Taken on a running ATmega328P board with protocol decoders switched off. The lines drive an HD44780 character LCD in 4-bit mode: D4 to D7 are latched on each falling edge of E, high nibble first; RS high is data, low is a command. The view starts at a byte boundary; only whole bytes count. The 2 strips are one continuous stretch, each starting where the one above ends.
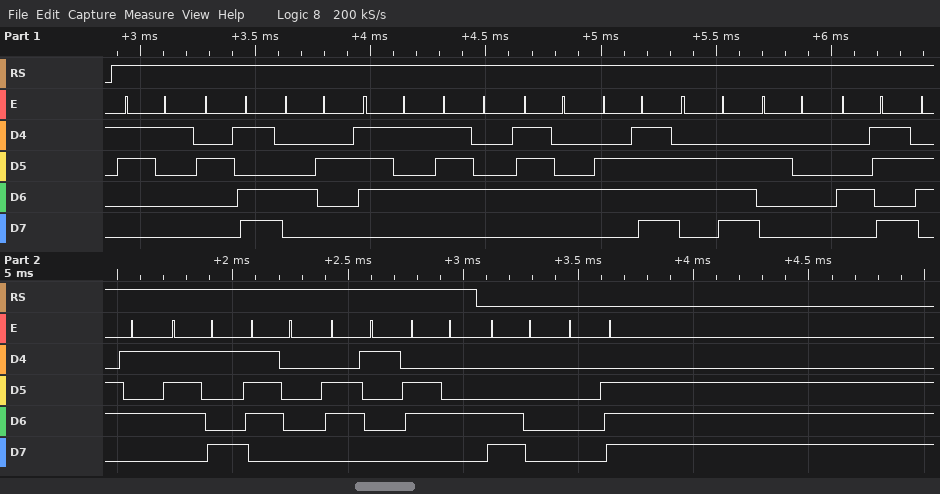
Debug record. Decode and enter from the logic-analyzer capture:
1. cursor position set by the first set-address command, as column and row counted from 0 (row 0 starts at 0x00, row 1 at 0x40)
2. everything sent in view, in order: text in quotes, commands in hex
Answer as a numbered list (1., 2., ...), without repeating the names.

1. column 0, row 1
2. "1-Button Keypad" 0xC0 0x0E
